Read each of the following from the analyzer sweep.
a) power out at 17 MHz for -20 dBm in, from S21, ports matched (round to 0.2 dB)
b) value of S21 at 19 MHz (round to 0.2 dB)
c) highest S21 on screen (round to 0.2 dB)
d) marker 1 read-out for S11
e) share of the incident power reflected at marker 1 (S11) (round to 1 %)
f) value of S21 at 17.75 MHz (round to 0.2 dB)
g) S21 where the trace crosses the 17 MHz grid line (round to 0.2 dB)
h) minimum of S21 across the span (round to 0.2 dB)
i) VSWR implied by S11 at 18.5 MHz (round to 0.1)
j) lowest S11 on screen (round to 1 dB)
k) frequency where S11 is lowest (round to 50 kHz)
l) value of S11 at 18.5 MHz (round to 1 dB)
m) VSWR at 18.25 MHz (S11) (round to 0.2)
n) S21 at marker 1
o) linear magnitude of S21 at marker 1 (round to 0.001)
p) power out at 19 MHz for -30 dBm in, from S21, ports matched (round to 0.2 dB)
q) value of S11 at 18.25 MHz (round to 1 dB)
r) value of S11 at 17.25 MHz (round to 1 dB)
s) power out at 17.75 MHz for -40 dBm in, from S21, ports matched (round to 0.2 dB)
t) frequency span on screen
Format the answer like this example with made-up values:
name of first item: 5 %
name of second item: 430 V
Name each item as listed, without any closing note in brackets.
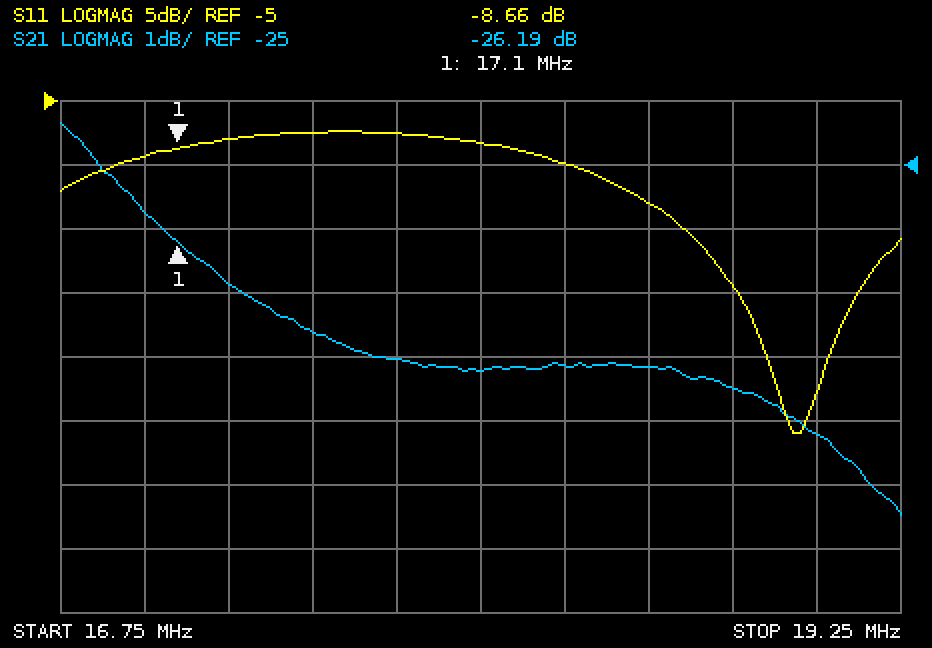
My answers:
power out at 17 MHz for -20 dBm in, from S21, ports matched: -45.8 dBm
value of S21 at 19 MHz: -29.2 dB
highest S21 on screen: -24.4 dB
marker 1 read-out for S11: -8.66 dB
share of the incident power reflected at marker 1 (S11): 14 %
value of S21 at 17.75 MHz: -28.0 dB
S21 where the trace crosses the 17 MHz grid line: -25.8 dB
minimum of S21 across the span: -30.4 dB
VSWR implied by S11 at 18.5 MHz: 1.6
lowest S11 on screen: -31 dB
frequency where S11 is lowest: 18.95 MHz
value of S11 at 18.5 MHz: -13 dB
VSWR at 18.25 MHz (S11): 2.0
S21 at marker 1: -26.19 dB
linear magnitude of S21 at marker 1: 0.049
power out at 19 MHz for -30 dBm in, from S21, ports matched: -59.2 dBm
value of S11 at 18.25 MHz: -10 dB
value of S11 at 17.25 MHz: -8 dB
power out at 17.75 MHz for -40 dBm in, from S21, ports matched: -68.0 dBm
frequency span on screen: 2.5 MHz
